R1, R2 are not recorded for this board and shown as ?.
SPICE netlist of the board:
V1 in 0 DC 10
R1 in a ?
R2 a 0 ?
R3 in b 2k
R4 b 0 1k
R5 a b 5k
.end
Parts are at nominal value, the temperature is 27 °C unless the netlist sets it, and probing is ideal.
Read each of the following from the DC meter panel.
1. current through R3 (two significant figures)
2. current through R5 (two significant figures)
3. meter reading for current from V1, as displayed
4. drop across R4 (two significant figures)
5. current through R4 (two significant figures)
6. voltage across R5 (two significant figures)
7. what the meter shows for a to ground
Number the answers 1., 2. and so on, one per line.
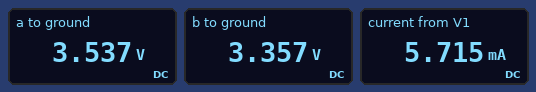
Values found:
1. 3.3 mA
2. 36 µA
3. 5.715 mA
4. 3.4 V
5. 3.4 mA
6. 180 mV
7. 3.537 V
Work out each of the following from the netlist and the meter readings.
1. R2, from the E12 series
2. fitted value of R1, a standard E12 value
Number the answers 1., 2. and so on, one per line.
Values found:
1. 1.5 kΩ
2. 2.7 kΩ
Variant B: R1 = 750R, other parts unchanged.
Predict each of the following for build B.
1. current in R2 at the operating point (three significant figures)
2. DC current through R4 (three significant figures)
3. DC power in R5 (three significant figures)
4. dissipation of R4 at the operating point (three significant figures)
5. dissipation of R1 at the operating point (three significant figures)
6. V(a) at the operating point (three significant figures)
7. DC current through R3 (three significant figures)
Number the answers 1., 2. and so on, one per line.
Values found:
1. 4.26 mA
2. 3.69 mA
3. 1.46 mW
4. 13.6 mW
5. 17.3 mW
6. 6.40 V
7. 3.15 mA
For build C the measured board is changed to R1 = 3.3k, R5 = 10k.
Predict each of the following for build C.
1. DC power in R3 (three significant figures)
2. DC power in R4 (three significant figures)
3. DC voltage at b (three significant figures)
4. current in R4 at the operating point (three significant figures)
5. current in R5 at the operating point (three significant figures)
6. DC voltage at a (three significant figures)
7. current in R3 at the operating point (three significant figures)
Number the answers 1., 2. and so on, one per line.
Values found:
1. 22.3 mW
2. 11.0 mW
3. 3.32 V
4. 3.32 mA
5. 17.8 µA
6. 3.14 V
7. 3.34 mA
